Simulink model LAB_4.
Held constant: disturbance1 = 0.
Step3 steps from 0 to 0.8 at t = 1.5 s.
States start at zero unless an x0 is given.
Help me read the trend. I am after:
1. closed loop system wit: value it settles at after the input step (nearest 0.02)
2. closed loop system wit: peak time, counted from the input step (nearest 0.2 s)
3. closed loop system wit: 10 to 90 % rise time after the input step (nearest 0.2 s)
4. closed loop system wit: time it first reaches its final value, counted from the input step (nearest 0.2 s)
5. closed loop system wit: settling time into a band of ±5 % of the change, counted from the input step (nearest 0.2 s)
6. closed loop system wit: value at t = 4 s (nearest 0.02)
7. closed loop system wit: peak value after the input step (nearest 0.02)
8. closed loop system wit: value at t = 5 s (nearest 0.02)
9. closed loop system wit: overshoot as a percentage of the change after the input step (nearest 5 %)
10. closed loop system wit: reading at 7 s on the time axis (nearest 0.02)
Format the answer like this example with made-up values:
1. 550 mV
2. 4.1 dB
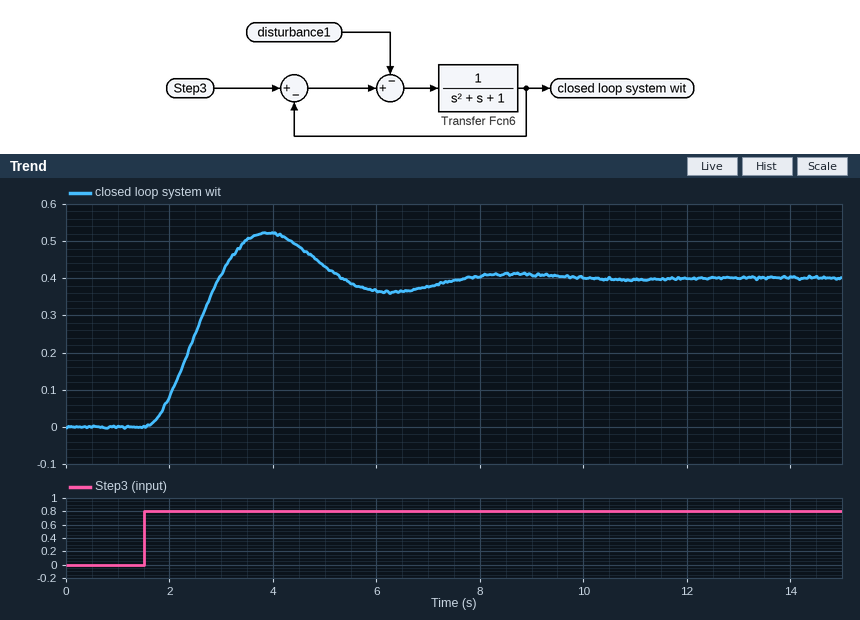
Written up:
1. 0.40
2. 2.4 s
3. 1.0 s
4. 1.4 s
5. 5.6 s
6. 0.52
7. 0.52
8. 0.44
9. 30 %
10. 0.38
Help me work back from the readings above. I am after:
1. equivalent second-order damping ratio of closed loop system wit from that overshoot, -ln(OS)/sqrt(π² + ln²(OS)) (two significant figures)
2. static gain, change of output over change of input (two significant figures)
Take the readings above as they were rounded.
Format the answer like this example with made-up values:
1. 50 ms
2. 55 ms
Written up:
1. 0.36
2. 0.50
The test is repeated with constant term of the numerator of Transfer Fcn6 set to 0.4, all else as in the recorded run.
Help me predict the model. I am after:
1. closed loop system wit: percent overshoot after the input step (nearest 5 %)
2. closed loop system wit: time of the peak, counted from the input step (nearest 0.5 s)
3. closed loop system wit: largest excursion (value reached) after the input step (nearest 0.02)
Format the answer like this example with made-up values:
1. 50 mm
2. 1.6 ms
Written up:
1. 25 %
2. 3.0 s
3. 0.28
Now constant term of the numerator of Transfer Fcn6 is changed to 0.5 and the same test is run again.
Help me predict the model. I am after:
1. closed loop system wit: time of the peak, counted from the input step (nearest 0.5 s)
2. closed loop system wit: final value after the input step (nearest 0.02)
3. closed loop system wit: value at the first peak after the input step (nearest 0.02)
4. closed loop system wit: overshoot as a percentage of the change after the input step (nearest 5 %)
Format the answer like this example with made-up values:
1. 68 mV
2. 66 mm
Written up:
1. 3.0 s
2. 0.26
3. 0.34
4. 25 %
